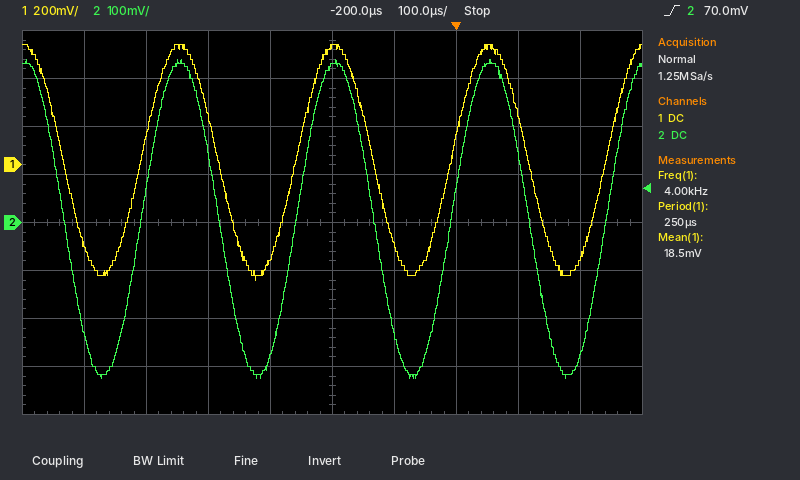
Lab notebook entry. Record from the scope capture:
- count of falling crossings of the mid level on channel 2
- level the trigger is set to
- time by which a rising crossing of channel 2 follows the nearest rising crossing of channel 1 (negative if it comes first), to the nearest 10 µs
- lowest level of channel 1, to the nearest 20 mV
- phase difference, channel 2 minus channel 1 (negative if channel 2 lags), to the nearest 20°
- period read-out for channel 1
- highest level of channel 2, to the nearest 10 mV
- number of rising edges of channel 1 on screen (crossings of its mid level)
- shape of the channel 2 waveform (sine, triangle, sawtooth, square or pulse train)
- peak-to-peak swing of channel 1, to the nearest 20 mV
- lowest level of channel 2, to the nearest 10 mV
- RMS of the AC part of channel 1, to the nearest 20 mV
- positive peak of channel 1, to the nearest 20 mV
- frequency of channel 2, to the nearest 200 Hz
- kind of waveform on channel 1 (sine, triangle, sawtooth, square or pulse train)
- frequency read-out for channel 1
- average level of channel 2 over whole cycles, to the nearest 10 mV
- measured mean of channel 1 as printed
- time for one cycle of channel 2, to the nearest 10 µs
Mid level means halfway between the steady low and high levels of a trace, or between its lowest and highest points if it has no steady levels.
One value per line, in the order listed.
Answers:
4
70.0 mV
0 µs
-480 mV
0°
250 µs
340 mV
4
sine
980 mV
-320 mV
340 mV
500 mV
4.0 kHz
sine
4.00 kHz
10 mV
18.5 mV
250 µs
